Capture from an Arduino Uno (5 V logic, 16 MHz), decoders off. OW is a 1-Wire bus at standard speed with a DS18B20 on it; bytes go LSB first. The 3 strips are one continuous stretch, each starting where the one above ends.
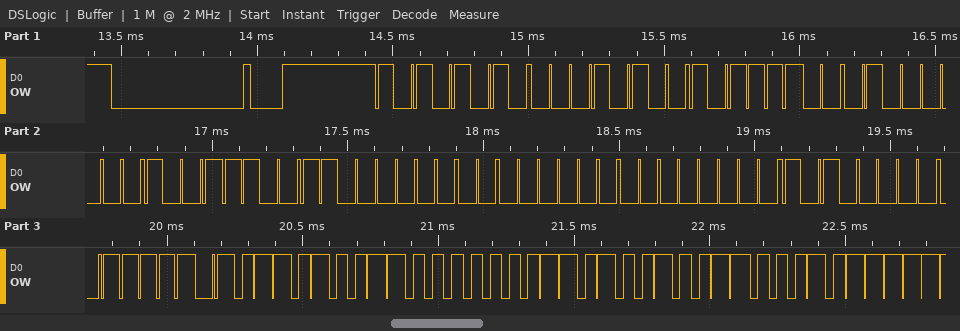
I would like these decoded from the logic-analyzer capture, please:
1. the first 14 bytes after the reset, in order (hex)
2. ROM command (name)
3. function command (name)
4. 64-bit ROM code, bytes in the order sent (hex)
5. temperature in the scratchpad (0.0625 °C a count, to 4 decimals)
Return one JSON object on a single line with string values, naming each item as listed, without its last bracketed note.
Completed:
{"the first 14 bytes after the reset, in order": "55 28 3D 02 39 03 00 00 05 BE 96 01 4B 46", "ROM command": "Match ROM", "function command": "Read Scratchpad", "64-bit ROM code, bytes in the order sent": "28 3D 02 39 03 00 00 05", "temperature in the scratchpad": "25.3750 °C"}
